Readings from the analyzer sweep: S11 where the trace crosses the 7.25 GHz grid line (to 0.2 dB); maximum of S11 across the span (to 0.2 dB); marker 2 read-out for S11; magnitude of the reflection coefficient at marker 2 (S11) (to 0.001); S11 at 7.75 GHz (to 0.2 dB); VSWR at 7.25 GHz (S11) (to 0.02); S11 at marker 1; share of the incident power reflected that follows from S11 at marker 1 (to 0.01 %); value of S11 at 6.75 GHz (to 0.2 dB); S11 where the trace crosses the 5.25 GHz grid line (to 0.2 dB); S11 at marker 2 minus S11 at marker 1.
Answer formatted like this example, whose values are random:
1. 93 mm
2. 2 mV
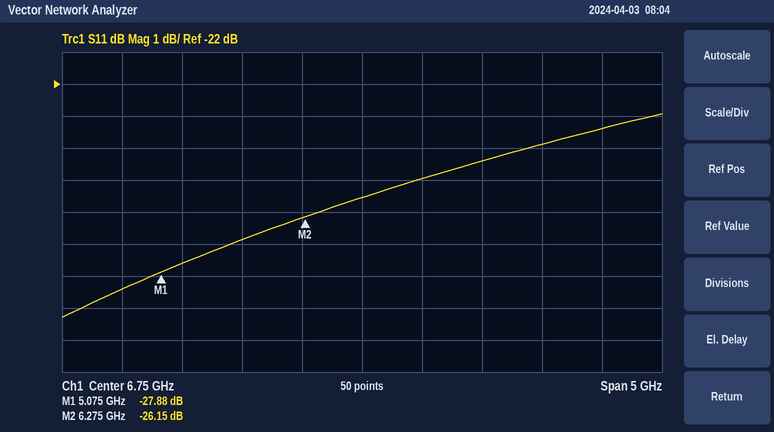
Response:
1. -25.0 dB
2. -23.0 dB
3. -26.15 dB
4. 0.049
5. -24.4 dB
6. 1.12
7. -27.88 dB
8. 0.16 %
9. -25.6 dB
10. -27.6 dB
11. 1.73 dB
